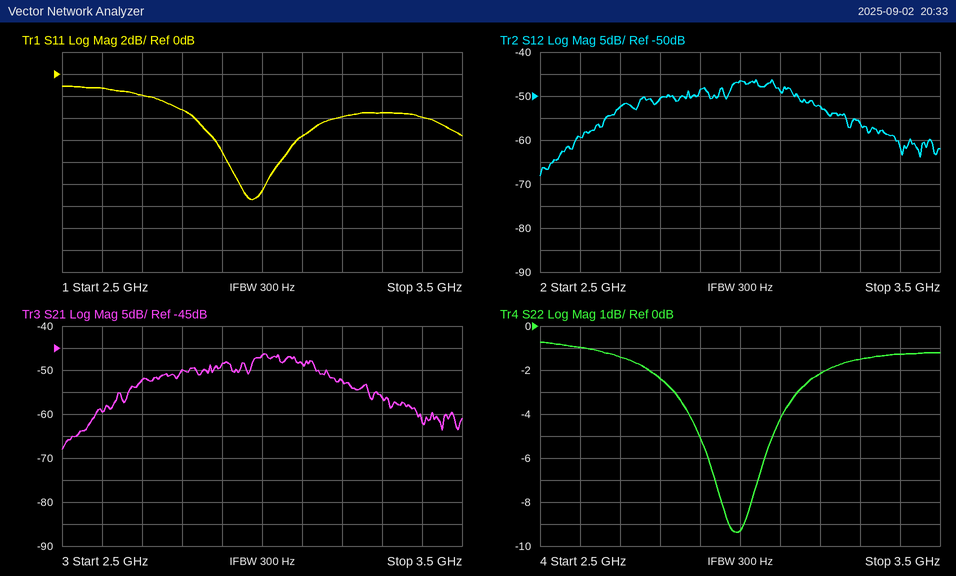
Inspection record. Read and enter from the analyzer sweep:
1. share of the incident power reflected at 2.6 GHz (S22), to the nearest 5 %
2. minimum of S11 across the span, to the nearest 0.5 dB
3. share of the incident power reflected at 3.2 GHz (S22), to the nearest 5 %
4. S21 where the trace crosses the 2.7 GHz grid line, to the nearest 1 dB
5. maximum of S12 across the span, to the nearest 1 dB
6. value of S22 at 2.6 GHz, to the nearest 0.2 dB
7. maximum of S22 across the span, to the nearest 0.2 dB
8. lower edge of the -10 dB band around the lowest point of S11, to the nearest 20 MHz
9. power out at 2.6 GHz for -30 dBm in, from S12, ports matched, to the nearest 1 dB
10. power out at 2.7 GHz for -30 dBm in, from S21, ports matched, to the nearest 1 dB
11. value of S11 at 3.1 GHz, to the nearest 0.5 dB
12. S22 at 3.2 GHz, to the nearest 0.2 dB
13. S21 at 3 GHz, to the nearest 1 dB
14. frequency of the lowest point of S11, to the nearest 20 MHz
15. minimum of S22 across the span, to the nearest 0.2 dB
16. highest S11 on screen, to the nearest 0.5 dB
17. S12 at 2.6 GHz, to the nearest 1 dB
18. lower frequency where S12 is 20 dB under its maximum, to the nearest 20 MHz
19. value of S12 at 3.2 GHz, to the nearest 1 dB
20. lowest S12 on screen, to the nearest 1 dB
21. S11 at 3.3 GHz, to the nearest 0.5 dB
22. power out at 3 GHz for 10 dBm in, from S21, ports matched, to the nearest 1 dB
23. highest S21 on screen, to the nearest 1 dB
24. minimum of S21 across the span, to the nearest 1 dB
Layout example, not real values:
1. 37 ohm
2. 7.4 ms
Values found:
1. 80 %
2. -11.5 dB
3. 60 %
4. -52 dB
5. -46 dB
6. -1.0 dB
7. -0.8 dB
8. 2.94 GHz
9. -89 dBm
10. -82 dBm
11. -5.5 dB
12. -2.2 dB
13. -47 dB
14. 2.98 GHz
15. -9.4 dB
16. -1.0 dB
17. -59 dB
18. 2.52 GHz
19. -52 dB
20. -68 dB
21. -3.5 dB
22. -37 dBm
23. -46 dB
24. -68 dB
